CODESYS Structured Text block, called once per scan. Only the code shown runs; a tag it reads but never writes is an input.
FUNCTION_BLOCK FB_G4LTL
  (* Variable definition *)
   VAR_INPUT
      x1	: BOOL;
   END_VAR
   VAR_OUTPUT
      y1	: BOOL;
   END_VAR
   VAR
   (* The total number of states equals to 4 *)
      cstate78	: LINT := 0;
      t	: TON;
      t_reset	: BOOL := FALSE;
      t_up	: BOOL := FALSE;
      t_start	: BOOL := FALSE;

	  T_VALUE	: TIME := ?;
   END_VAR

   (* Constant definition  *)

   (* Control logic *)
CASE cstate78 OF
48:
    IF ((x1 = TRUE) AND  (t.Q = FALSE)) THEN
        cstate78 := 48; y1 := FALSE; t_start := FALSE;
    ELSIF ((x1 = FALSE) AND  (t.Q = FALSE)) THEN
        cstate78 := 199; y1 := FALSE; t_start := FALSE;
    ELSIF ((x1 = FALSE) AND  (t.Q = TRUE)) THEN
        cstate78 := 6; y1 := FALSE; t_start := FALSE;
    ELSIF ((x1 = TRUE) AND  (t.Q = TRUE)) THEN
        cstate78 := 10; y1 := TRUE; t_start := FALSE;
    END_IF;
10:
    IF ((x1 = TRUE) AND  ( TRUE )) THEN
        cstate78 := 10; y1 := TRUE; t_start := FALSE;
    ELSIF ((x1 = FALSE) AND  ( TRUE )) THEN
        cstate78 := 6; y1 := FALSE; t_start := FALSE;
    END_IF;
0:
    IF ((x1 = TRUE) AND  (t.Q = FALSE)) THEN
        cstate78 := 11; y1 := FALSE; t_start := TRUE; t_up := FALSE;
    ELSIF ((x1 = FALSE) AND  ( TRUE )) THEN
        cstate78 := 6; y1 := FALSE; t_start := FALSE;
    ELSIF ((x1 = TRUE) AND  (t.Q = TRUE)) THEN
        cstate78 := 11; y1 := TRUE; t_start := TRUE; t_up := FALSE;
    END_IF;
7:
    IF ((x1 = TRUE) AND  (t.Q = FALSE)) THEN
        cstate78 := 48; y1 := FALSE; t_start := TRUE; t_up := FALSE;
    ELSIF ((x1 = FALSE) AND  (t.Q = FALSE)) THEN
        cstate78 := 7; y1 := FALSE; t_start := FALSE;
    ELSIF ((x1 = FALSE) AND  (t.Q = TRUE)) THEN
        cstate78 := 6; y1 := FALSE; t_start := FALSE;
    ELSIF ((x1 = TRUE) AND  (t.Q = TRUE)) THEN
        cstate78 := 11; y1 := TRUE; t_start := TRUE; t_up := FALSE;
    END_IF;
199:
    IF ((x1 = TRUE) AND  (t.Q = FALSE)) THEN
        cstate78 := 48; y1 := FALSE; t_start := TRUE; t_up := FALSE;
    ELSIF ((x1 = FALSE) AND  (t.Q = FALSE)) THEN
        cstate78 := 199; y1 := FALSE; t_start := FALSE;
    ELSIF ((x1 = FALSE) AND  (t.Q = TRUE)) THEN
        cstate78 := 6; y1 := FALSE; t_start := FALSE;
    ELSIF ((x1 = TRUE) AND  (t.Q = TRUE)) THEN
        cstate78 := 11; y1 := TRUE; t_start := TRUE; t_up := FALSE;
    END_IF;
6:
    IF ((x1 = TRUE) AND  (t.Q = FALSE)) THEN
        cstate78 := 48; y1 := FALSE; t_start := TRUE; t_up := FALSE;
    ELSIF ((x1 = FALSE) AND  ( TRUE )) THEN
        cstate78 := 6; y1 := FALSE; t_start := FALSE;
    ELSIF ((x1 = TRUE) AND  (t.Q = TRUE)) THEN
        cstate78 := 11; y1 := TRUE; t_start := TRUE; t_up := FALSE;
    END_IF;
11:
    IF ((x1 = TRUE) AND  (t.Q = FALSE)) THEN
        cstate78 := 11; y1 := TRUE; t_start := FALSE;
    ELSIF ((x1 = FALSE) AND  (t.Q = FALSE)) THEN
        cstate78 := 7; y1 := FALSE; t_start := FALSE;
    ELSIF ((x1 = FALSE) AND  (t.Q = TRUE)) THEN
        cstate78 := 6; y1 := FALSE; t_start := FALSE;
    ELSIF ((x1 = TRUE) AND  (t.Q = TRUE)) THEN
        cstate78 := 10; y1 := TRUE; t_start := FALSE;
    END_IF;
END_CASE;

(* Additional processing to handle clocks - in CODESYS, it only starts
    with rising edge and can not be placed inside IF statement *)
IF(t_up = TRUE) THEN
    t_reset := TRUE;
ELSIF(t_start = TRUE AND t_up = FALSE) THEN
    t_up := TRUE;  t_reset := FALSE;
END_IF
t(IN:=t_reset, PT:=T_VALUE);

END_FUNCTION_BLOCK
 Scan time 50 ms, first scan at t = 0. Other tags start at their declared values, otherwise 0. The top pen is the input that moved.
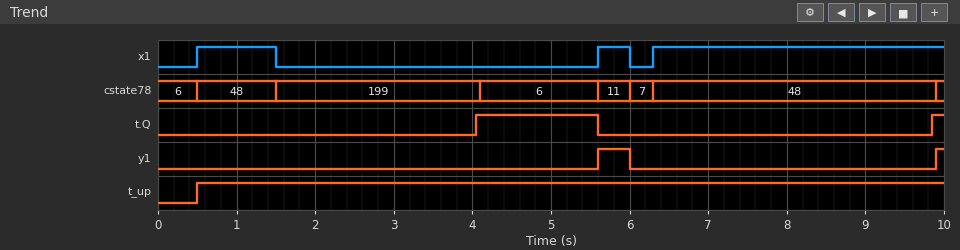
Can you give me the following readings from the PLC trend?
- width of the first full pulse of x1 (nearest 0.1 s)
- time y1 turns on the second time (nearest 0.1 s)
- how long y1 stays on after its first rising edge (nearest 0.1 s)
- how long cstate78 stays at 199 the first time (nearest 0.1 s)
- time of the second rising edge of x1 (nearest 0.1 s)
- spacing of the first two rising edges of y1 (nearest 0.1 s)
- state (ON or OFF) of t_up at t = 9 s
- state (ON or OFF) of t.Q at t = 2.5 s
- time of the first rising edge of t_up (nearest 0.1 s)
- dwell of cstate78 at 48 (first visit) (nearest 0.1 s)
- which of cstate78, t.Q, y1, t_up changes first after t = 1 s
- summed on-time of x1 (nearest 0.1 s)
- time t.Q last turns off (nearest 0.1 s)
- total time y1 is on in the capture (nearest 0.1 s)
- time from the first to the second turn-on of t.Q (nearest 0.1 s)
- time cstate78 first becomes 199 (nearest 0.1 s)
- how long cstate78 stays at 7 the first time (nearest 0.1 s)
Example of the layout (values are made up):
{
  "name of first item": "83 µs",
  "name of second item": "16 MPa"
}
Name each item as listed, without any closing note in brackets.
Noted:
{
  "width of the first full pulse of x1": "1.0 s",
  "time y1 turns on the second time": "9.9 s",
  "how long y1 stays on after its first rising edge": "0.4 s",
  "how long cstate78 stays at 199 the first time": "2.6 s",
  "time of the second rising edge of x1": "5.6 s",
  "spacing of the first two rising edges of y1": "4.3 s",
  "state (ON or OFF) of t_up at t = 9 s": "ON",
  "state (ON or OFF) of t.Q at t = 2.5 s": "OFF",
  "time of the first rising edge of t_up": "0.5 s",
  "dwell of cstate78 at 48 (first visit)": "1.0 s",
  "which of cstate78, t.Q, y1, t_up changes first after t = 1 s": "cstate78",
  "summed on-time of x1": "5.1 s",
  "time t.Q last turns off": "5.6 s",
  "total time y1 is on in the capture": "0.5 s",
  "time from the first to the second turn-on of t.Q": "5.8 s",
  "time cstate78 first becomes 199": "1.5 s",
  "how long cstate78 stays at 7 the first time": "0.3 s"
}
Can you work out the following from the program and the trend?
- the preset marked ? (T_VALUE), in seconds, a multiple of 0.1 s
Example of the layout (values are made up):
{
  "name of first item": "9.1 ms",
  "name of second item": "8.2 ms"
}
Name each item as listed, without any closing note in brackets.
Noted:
{
  "the preset marked ? (T_VALUE), in seconds, a multiple of 0.1 s": "3.5 s"
}
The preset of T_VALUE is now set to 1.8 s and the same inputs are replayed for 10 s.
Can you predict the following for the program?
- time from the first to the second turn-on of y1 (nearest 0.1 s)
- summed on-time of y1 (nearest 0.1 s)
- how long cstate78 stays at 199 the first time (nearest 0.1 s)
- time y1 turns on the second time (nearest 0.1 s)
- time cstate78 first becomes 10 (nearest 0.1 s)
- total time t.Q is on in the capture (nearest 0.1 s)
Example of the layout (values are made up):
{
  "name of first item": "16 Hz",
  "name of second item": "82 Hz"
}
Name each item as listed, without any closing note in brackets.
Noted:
{
  "time from the first to the second turn-on of y1": "2.6 s",
  "summed on-time of y1": "2.2 s",
  "how long cstate78 stays at 199 the first time": "0.9 s",
  "time y1 turns on the second time": "8.2 s",
  "time cstate78 first becomes 10": "8.2 s",
  "total time t.Q is on in the capture": "5.1 s"
}
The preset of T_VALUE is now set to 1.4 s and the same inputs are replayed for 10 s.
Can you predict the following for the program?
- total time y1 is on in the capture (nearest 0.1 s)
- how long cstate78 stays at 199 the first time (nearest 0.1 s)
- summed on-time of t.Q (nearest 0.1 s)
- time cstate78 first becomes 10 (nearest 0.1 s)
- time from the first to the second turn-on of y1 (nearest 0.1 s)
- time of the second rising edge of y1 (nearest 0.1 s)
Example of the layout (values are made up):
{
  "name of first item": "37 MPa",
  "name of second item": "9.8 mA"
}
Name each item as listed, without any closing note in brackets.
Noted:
{
  "total time y1 is on in the capture": "2.6 s",
  "how long cstate78 stays at 199 the first time": "0.5 s",
  "summed on-time of t.Q": "5.9 s",
  "time cstate78 first becomes 10": "7.8 s",
  "time from the first to the second turn-on of y1": "2.2 s",
  "time of the second rising edge of y1": "7.8 s"
}
